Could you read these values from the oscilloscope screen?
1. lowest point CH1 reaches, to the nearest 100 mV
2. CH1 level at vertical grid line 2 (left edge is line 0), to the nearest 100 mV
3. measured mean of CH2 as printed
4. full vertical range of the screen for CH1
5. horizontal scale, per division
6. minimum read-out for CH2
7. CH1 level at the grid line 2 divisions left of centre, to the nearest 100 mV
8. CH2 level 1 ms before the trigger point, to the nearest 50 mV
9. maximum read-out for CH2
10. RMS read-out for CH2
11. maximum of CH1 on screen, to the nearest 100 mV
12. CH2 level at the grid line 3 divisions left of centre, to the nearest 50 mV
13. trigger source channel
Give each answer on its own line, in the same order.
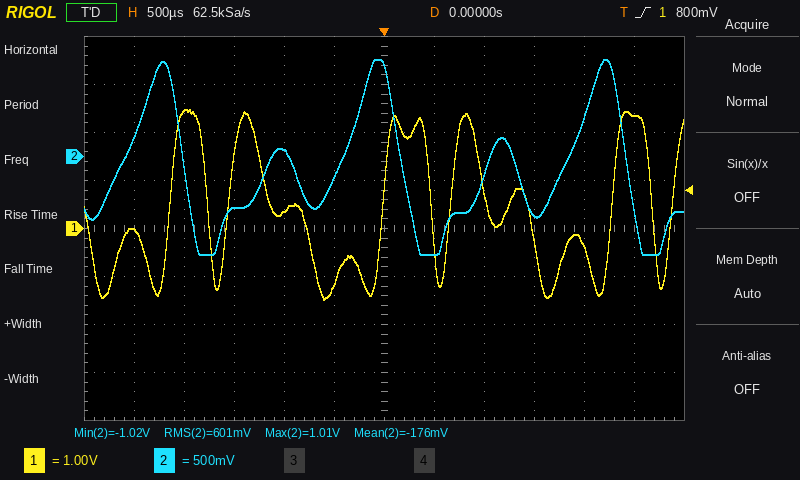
-1.5 V
2.4 V
-176 mV
8 V
500 µs
-1.02 V
300 mV
50 mV
1.01 V
601 mV
2.5 V
-550 mV
CH1
